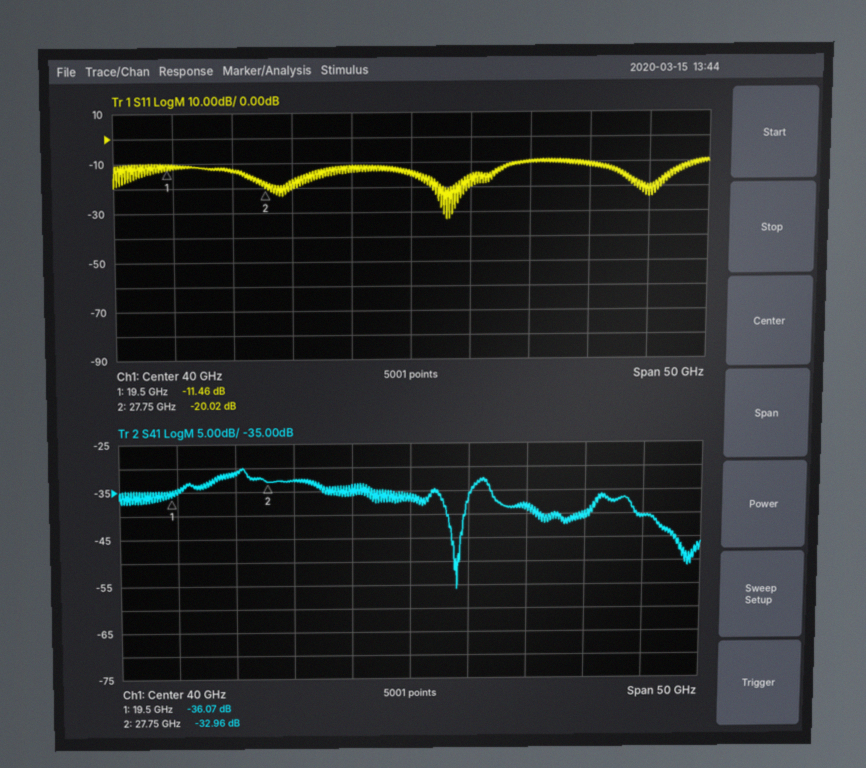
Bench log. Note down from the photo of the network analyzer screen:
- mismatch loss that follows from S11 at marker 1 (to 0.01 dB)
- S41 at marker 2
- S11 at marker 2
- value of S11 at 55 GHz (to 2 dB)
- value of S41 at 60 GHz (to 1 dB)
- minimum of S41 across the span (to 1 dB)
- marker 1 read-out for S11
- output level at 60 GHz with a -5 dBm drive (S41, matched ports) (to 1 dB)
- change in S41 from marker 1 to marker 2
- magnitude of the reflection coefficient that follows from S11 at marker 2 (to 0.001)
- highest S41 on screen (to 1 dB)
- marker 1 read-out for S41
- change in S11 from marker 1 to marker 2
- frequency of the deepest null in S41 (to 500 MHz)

0.32 dB
-32.96 dB
-20.02 dB
-12 dB
-41 dB
-56 dB
-11.46 dB
-46 dBm
3.11 dB
0.100
-30 dB
-36.07 dB
-8.56 dB
44.0 GHz
